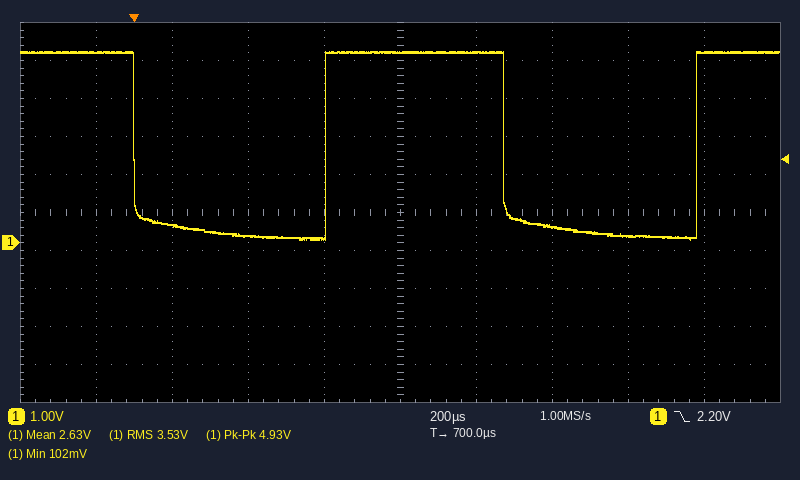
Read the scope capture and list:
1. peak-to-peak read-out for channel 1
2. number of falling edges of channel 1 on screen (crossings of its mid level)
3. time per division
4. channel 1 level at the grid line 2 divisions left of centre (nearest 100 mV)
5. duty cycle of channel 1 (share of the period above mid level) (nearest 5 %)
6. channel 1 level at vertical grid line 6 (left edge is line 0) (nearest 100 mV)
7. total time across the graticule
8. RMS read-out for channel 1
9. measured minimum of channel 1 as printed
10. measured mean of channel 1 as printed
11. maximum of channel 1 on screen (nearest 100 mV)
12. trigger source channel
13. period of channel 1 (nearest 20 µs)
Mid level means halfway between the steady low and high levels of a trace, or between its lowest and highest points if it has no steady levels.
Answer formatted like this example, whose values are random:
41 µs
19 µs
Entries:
4.93 V
2
200 µs
200 mV
50 %
5.0 V
2 ms
3.53 V
102 mV
2.63 V
5.0 V
channel 1
980 µs
